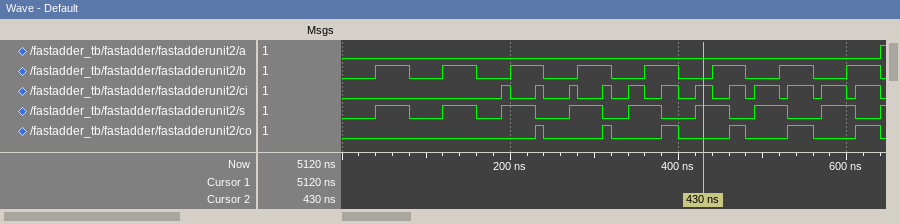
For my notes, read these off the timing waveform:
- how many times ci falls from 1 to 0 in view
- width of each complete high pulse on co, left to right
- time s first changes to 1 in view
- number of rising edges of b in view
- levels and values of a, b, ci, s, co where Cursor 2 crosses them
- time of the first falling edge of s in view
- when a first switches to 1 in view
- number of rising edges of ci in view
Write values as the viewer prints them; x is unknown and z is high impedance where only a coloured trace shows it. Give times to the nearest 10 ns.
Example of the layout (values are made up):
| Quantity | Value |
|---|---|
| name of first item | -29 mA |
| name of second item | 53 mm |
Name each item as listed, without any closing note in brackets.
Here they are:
| Quantity | Value |
|---|---|
| how many times ci falls from 1 to 0 in view | 12 |
| width of each complete high pulse on co, left to right | 10 ns, 10 ns, 20 ns, 20 ns, 30 ns, 30 ns |
| time s first changes to 1 in view | 40 ns |
| number of rising edges of b in view | 8 |
| levels and values of a, b, ci, s, co where Cursor 2 crosses them | a=0, b=0, ci=1, s=1, co=0 |
| time of the first falling edge of s in view | 80 ns |
| when a first switches to 1 in view | 640 ns |
| number of rising edges of ci in view | 12 |
